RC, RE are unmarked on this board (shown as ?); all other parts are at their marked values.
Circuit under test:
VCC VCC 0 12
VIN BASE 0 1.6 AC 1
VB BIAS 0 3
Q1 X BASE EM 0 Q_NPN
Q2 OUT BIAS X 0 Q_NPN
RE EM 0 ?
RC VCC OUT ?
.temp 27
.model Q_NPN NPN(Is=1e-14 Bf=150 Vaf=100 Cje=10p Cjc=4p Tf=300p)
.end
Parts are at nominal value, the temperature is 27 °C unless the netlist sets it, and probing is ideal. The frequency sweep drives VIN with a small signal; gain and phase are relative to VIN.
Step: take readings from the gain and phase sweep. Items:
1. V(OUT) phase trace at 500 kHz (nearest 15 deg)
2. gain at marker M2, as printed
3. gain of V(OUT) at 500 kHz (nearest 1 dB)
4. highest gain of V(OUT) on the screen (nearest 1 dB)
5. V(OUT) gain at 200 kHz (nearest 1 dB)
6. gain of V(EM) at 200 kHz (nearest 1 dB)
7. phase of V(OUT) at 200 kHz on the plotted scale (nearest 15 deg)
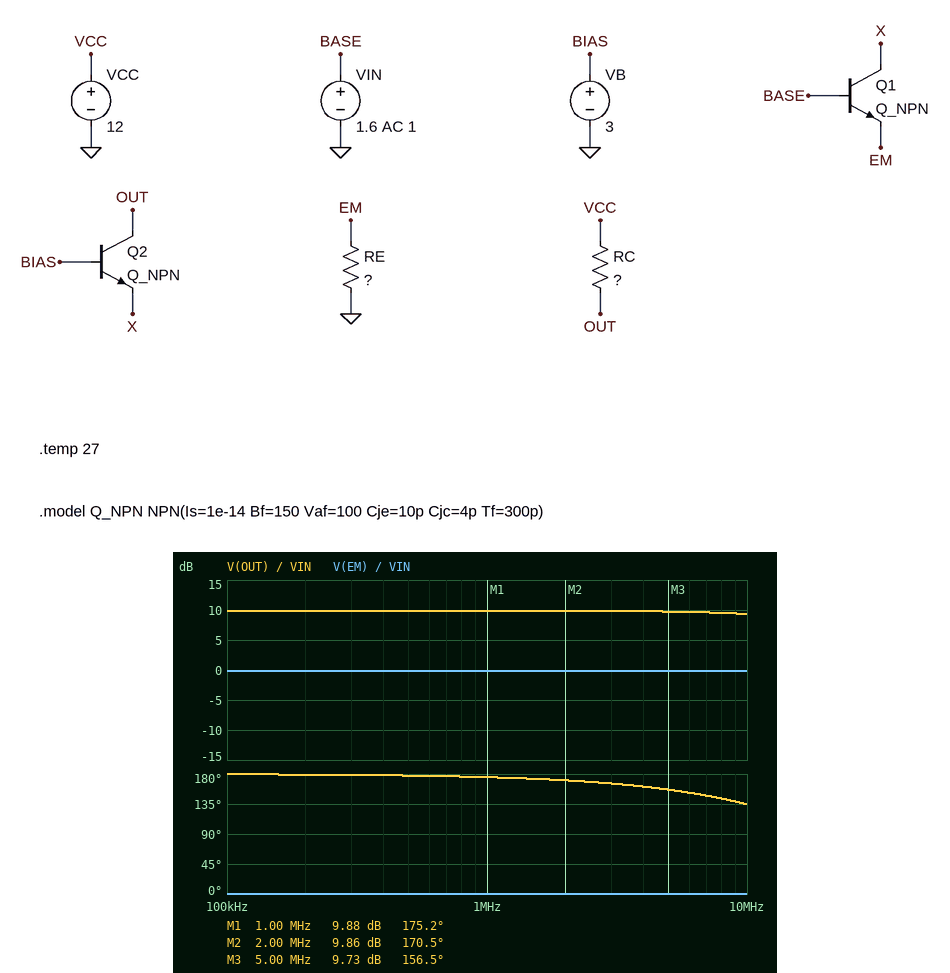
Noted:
180 deg
9.86 dB
10 dB
10 dB
10 dB
0 dB
180 deg
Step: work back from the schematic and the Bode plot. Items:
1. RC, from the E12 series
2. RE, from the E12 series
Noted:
3.9 kΩ
1.2 kΩ
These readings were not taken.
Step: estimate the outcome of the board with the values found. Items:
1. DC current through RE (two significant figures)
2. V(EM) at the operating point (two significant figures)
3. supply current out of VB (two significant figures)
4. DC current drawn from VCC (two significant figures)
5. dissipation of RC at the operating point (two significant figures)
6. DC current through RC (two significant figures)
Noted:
790 µA
950 mV
4.9 µA
780 µA
2.4 mW
780 µA
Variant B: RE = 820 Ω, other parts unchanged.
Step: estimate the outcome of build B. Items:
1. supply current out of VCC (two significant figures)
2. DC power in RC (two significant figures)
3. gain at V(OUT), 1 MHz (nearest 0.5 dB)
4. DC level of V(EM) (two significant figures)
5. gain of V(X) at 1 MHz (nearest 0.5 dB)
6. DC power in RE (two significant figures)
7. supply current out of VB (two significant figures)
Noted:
1.1 mA
5.0 mW
13.0 dB
940 mV
-31.0 dB
1.1 mW
7.2 µA
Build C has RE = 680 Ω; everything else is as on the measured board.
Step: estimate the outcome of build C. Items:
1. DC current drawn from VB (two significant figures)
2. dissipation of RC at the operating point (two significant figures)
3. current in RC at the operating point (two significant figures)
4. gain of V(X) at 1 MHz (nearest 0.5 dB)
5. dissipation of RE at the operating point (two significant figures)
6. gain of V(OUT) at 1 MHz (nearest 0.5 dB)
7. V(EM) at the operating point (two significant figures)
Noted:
8.7 µA
7.2 mW
1.4 mA
-31.0 dB
1.3 mW
15.0 dB
940 mV
